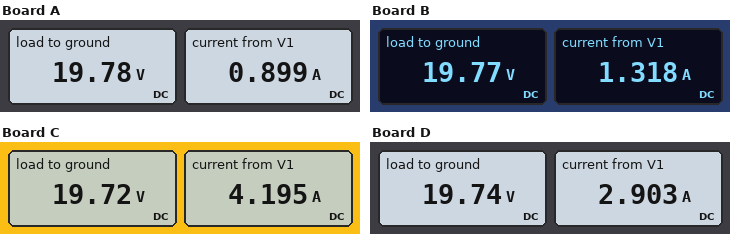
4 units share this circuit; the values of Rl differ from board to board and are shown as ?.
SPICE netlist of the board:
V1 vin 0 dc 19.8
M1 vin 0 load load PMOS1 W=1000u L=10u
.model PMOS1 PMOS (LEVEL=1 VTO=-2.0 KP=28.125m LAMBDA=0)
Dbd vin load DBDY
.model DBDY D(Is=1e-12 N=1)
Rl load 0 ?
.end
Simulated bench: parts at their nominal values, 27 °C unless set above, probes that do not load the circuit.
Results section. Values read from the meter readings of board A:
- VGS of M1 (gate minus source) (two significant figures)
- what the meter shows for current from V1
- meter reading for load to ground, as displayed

-20 V
0.899 A
19.78 V
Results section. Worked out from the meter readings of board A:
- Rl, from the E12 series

22 Ω
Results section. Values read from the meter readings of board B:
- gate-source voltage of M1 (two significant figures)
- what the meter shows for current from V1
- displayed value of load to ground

-20 V
1.318 A
19.77 V
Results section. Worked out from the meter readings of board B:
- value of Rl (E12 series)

15 Ω
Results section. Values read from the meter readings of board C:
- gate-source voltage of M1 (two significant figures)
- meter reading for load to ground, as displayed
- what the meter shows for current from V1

-20 V
19.72 V
4.195 A
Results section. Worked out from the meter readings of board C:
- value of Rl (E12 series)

4.7 Ω
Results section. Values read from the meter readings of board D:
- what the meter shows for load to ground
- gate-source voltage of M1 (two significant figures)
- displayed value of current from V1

19.74 V
-20 V
2.903 A
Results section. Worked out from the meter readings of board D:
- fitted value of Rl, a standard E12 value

6.8 Ω
